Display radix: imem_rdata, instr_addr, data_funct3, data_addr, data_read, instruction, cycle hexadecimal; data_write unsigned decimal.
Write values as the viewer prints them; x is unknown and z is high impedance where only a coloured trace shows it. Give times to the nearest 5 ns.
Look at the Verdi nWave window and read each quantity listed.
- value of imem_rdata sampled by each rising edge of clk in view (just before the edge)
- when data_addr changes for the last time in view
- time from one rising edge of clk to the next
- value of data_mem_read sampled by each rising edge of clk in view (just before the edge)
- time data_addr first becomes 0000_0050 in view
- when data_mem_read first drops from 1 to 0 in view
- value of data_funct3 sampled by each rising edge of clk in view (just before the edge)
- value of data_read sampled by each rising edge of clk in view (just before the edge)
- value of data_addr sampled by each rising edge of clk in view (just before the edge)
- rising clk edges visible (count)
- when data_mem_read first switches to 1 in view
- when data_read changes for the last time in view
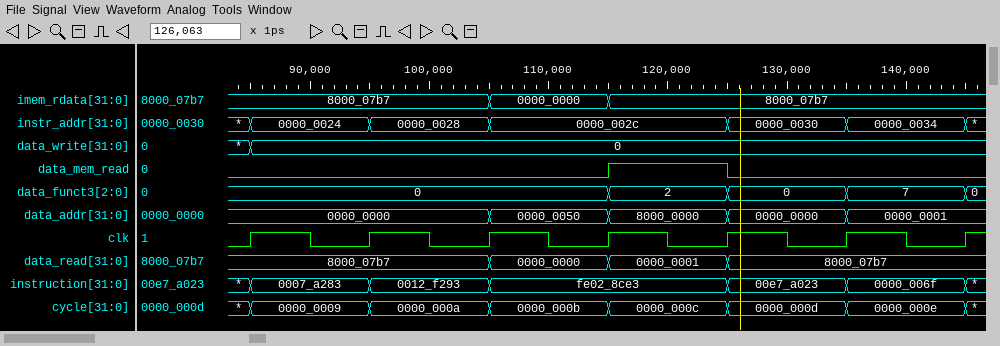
8000_07b7, 8000_07b7, 8000_07b7, 0000_0000, 8000_07b7, 8000_07b7, 8000_07b7
135 ns
10 ns
0 0 0 0 1 0 0
105 ns
125 ns
0, 0, 0, 0, 2, 0, 7
8000_07b7, 8000_07b7, 8000_07b7, 0000_0000, 0000_0001, 8000_07b7, 8000_07b7
0000_0000, 0000_0000, 0000_0000, 0000_0050, 8000_0000, 0000_0000, 0000_0001
7
115 ns
125 ns
